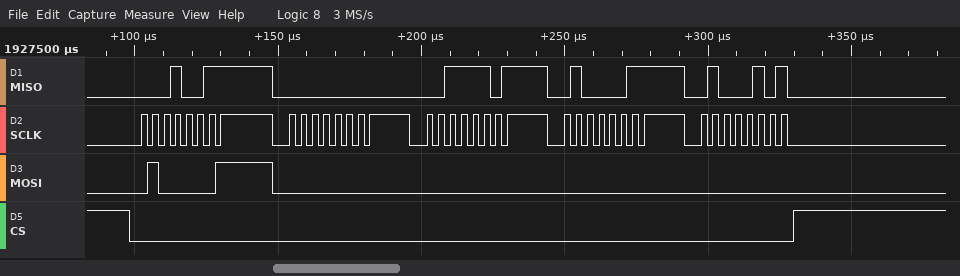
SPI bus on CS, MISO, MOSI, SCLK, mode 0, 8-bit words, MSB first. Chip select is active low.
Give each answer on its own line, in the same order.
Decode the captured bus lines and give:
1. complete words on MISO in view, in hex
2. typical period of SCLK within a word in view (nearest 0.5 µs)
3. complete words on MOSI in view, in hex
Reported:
13, 00, 3D, 43, 45
4 µs
41, 00, 00, 00, 00
